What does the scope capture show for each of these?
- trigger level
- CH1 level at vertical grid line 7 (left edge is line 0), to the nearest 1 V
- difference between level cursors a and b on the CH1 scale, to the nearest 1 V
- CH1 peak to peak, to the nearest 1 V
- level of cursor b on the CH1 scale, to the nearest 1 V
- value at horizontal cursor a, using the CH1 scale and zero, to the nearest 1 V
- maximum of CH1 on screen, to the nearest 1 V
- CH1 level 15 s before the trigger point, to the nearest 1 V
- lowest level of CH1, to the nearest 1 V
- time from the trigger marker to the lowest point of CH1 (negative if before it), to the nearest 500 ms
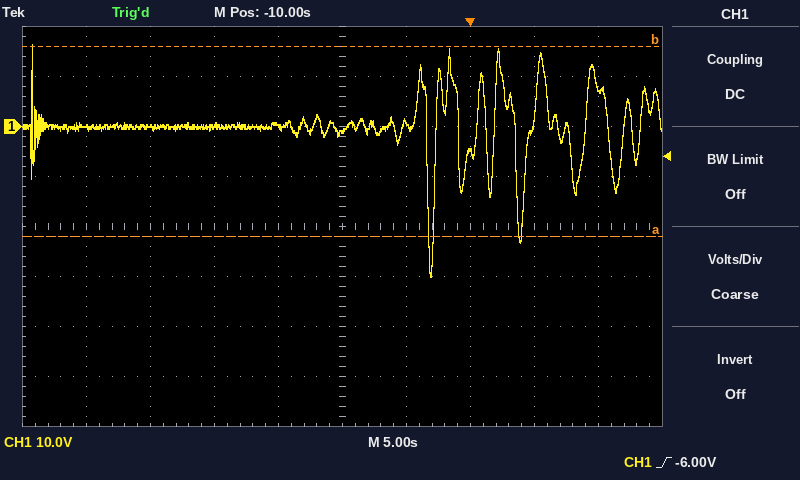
-6.00 V
-5 V
38 V
46 V
16 V
-22 V
16 V
0 V
-30 V
-3.0 s
